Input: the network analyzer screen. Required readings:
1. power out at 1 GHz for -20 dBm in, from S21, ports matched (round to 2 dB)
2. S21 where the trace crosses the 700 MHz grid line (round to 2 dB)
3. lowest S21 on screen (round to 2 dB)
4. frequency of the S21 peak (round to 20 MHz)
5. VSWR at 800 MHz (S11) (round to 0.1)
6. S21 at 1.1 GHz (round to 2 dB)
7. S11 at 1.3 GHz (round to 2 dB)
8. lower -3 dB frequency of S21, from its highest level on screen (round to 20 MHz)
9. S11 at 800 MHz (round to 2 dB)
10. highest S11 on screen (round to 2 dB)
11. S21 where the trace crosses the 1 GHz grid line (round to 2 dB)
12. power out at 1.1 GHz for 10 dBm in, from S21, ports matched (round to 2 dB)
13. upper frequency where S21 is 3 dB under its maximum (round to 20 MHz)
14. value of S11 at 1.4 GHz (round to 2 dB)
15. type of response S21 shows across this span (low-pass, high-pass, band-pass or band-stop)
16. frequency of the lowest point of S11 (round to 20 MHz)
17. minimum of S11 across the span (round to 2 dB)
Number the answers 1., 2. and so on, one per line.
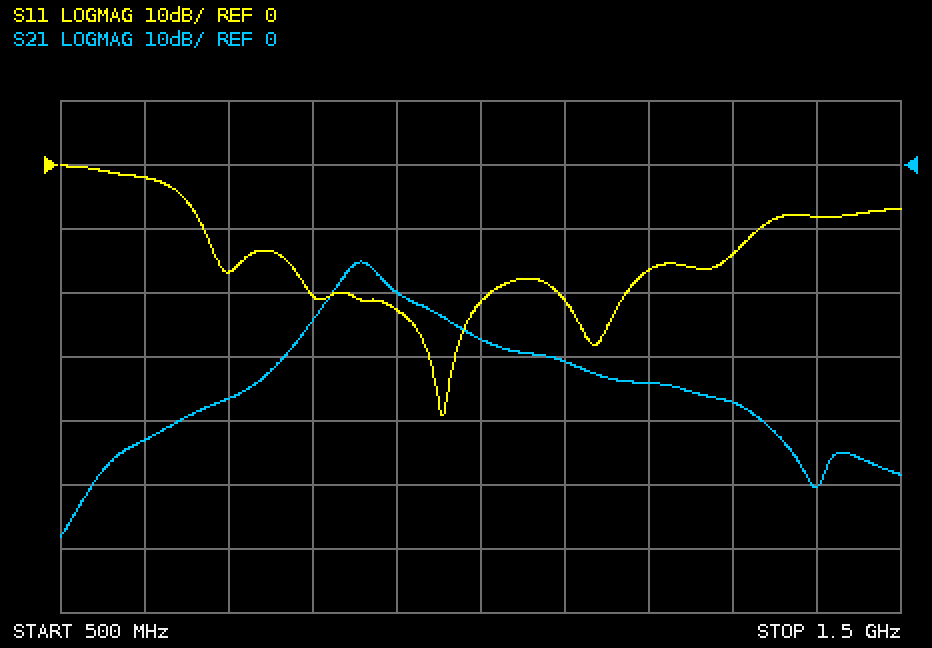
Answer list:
1. -48 dBm
2. -36 dB
3. -58 dB
4. 860 MHz
5. 1.2
6. -30 dB
7. -14 dB
8. 840 MHz
9. -20 dB
10. 0 dB
11. -28 dB
12. -20 dBm
13. 880 MHz
14. -8 dB
15. band-pass
16. 960 MHz
17. -40 dB
